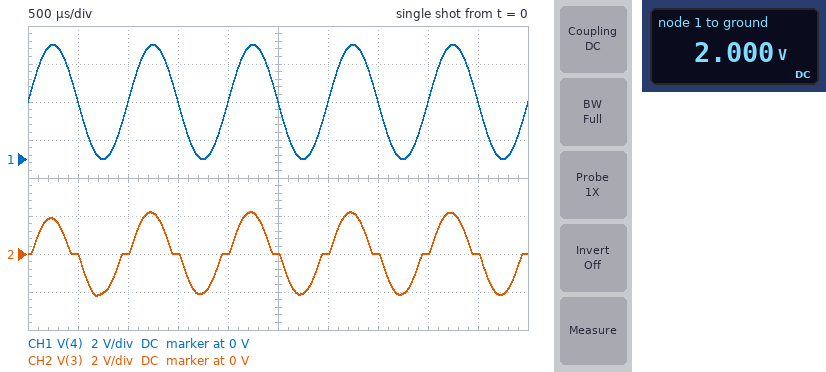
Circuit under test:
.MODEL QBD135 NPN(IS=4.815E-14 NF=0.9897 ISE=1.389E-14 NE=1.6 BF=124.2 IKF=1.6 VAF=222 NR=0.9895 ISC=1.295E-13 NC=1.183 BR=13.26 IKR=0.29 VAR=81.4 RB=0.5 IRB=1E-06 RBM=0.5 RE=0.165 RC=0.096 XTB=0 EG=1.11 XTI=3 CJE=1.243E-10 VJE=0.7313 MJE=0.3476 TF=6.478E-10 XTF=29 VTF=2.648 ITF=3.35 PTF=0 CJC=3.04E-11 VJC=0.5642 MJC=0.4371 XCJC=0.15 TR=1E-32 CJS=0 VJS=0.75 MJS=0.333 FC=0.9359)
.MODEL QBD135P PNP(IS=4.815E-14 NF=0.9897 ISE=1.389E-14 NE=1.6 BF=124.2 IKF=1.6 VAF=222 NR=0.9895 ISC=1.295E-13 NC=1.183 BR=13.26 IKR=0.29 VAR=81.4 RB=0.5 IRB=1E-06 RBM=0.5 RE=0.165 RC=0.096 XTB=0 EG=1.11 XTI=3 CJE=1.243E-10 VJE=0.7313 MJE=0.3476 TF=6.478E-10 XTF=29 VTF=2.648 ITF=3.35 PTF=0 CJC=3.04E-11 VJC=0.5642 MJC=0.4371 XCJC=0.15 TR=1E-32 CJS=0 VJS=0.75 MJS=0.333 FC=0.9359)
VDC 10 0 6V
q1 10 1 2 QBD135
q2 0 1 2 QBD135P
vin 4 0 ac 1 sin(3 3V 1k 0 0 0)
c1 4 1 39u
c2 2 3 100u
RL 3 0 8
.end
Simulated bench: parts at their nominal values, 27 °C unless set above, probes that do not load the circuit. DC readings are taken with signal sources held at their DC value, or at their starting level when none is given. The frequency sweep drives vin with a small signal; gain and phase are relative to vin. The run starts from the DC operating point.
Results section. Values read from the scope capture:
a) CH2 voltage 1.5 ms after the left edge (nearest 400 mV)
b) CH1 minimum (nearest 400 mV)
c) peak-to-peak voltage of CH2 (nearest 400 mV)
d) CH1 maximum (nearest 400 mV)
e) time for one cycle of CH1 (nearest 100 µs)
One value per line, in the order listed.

0 V
0 V
4.4 V
6.0 V
1.0 ms
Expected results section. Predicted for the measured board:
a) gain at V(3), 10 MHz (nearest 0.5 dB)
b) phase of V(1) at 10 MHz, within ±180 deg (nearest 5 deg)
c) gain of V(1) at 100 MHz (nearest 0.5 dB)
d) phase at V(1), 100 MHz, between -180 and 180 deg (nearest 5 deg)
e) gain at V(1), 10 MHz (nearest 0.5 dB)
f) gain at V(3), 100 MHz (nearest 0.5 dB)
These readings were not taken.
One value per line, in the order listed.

-18.0 dB
0 deg
0 dB
0 deg
0 dB
-2.5 dB
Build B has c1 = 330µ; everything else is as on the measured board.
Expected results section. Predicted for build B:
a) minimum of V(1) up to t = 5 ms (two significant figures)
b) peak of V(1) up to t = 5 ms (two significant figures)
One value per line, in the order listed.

-960 mV
5.2 V
